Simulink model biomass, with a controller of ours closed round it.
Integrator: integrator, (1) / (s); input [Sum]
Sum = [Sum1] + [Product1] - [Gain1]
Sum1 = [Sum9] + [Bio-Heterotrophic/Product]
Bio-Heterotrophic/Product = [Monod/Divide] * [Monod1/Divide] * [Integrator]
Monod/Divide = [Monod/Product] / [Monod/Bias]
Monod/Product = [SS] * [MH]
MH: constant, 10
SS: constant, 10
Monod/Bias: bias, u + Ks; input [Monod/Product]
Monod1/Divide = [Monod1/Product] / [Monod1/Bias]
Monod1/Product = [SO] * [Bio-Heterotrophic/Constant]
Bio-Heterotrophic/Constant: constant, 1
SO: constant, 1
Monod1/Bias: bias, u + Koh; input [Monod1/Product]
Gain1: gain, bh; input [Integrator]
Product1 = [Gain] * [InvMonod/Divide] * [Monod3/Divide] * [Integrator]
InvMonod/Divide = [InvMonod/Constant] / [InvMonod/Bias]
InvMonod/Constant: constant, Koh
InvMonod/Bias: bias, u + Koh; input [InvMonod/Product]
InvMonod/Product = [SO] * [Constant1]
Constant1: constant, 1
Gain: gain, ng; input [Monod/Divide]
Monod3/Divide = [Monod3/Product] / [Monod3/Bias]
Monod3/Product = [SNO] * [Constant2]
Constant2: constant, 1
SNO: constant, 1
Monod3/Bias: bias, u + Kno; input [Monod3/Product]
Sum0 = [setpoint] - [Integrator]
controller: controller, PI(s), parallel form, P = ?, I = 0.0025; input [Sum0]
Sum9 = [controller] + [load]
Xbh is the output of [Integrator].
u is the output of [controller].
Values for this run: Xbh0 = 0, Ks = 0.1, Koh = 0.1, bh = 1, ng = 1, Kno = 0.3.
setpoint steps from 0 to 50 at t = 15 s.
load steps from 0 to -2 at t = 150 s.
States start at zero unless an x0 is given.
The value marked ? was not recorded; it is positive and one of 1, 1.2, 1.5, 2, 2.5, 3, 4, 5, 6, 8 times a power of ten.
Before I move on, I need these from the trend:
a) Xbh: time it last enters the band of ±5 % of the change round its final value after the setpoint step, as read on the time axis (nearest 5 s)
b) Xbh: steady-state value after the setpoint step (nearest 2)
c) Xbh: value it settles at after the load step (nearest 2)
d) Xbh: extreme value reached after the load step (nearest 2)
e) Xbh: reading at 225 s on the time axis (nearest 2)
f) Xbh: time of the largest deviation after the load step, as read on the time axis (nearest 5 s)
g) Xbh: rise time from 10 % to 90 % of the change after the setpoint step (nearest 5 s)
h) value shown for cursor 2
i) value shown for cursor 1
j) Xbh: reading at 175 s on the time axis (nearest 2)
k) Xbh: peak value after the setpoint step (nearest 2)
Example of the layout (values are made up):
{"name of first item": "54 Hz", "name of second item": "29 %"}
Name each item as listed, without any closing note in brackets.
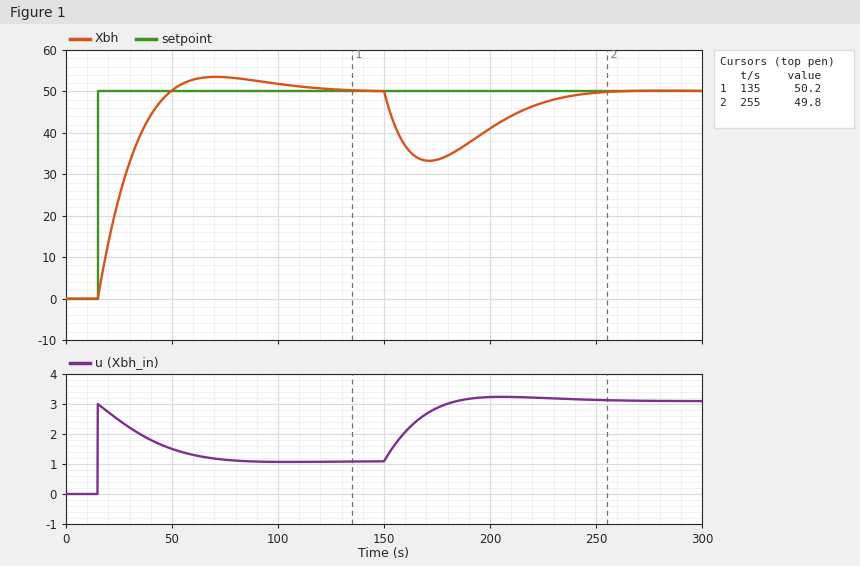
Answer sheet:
{"Xbh: time it last enters the band of ±5 % of the change round its final value after the setpoint step, as read on the time axis": "90 s", "Xbh: steady-state value after the setpoint step": "50", "Xbh: value it settles at after the load step": "50", "Xbh: extreme value reached after the load step": "34", "Xbh: reading at 225 s on the time axis": "48", "Xbh: time of the largest deviation after the load step, as read on the time axis": "170 s", "Xbh: rise time from 10 % to 90 % of the change after the setpoint step": "25 s", "value shown for cursor 2": "49.8", "value shown for cursor 1": "50.2", "Xbh: reading at 175 s on the time axis": "34", "Xbh: peak value after the setpoint step": "54"}
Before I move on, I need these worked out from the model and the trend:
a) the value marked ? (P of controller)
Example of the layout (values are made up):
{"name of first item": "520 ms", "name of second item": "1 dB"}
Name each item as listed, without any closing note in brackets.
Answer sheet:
{"the value marked ?": "0.06"}
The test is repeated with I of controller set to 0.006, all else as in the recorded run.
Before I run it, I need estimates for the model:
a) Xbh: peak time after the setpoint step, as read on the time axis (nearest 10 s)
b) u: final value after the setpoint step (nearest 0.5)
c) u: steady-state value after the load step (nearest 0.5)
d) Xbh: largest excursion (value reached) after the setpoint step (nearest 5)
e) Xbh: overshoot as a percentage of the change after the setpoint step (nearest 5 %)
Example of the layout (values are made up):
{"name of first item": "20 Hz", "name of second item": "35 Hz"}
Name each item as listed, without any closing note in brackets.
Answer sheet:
{"Xbh: peak time after the setpoint step, as read on the time axis": "50 s", "u: final value after the setpoint step": "1.0", "u: steady-state value after the load step": "3.0", "Xbh: largest excursion (value reached) after the setpoint step": "60", "Xbh: overshoot as a percentage of the change after the setpoint step": "20 %"}
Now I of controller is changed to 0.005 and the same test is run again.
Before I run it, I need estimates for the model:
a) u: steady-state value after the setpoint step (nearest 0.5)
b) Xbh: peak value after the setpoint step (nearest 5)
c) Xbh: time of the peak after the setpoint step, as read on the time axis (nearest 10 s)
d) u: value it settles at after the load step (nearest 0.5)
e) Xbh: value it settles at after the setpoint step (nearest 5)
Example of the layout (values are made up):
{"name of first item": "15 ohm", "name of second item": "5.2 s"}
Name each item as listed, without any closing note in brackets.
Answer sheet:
{"u: steady-state value after the setpoint step": "1.0", "Xbh: peak value after the setpoint step": "60", "Xbh: time of the peak after the setpoint step, as read on the time axis": "50 s", "u: value it settles at after the load step": "3.0", "Xbh: value it settles at after the setpoint step": "50"}
